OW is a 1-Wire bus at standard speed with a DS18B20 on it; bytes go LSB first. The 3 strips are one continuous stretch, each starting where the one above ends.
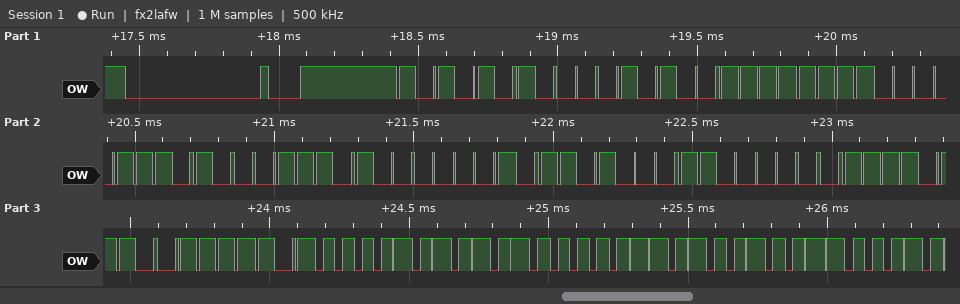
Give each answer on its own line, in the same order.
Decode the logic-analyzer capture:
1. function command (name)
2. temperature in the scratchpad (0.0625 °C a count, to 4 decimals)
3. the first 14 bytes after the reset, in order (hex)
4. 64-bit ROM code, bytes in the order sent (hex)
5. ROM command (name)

Read Scratchpad
85.0000 °C
55 28 FF 70 71 81 16 03 6F BE 50 05 4B 46
28 FF 70 71 81 16 03 6F
Match ROM
